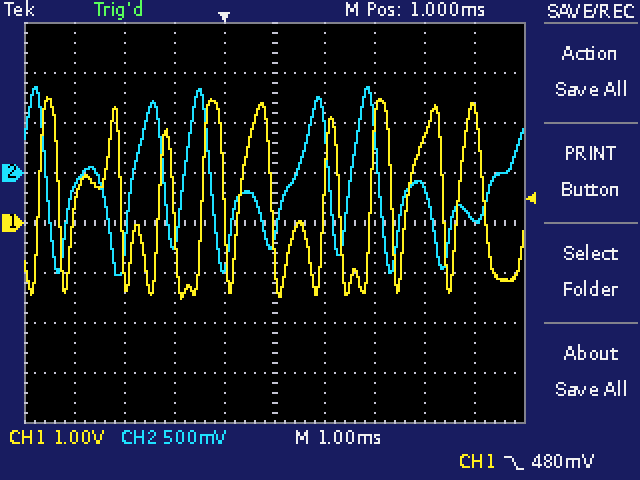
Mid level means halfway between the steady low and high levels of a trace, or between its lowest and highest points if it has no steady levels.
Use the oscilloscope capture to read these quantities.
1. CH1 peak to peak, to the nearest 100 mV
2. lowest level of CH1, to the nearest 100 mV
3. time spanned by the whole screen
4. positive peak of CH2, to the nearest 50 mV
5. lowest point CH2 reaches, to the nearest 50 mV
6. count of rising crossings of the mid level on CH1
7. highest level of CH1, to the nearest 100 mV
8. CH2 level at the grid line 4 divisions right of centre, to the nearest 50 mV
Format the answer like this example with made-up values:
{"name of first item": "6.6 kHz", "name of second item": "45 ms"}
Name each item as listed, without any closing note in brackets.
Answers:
{"CH1 peak to peak, to the nearest 100 mV": "4.0 V", "lowest level of CH1, to the nearest 100 mV": "-1.5 V", "time spanned by the whole screen": "10 ms", "positive peak of CH2, to the nearest 50 mV": "850 mV", "lowest point CH2 reaches, to the nearest 50 mV": "-1.00 V", "count of rising crossings of the mid level on CH1": "9", "highest level of CH1, to the nearest 100 mV": "2.5 V", "CH2 level at the grid line 4 divisions right of centre, to the nearest 50 mV": "-450 mV"}
